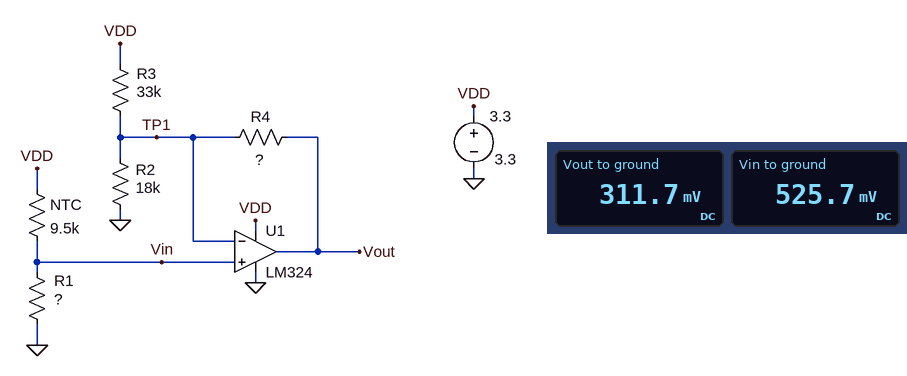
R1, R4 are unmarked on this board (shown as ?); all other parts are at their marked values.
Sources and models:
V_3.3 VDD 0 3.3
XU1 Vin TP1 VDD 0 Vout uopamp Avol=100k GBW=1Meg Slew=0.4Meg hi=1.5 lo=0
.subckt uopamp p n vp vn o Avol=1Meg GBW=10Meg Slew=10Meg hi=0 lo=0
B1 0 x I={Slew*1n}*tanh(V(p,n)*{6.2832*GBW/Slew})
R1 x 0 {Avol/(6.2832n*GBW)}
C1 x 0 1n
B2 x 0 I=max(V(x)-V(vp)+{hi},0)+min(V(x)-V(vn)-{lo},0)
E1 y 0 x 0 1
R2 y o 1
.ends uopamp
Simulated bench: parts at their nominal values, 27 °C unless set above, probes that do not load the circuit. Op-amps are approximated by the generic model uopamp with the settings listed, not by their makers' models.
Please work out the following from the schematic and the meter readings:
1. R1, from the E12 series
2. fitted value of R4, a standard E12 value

1.8 kΩ
3.9 kΩ
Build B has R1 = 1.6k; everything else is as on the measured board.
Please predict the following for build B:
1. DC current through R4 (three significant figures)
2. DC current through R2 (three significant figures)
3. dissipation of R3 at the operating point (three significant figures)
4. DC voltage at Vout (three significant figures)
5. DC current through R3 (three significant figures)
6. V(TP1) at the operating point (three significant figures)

59.2 µA
26.4 µA
242 µW
245 mV
85.6 µA
476 mV
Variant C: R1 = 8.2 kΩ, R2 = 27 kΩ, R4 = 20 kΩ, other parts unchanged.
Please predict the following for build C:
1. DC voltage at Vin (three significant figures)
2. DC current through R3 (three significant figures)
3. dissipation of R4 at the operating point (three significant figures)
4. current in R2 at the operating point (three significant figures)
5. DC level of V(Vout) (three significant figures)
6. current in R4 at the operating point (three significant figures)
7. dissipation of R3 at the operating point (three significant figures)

1.53 V
53.7 µA
174 nW
56.6 µA
1.59 V
2.95 µA
95.1 µW
